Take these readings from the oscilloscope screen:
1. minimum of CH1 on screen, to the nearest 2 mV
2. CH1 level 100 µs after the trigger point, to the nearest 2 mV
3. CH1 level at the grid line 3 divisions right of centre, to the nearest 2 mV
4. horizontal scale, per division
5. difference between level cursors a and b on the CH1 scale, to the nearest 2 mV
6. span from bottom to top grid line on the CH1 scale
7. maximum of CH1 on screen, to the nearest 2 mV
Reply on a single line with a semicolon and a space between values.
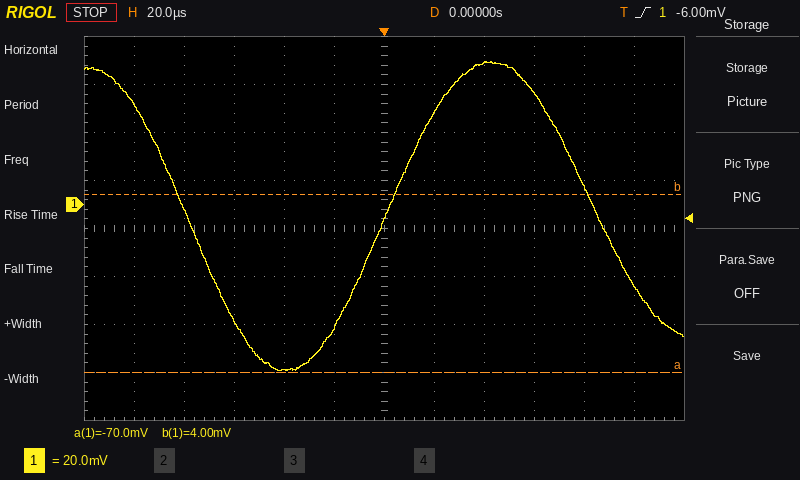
-70 mV; -34 mV; 46 mV; 20 µs; 74 mV; 160 mV; 60 mV
